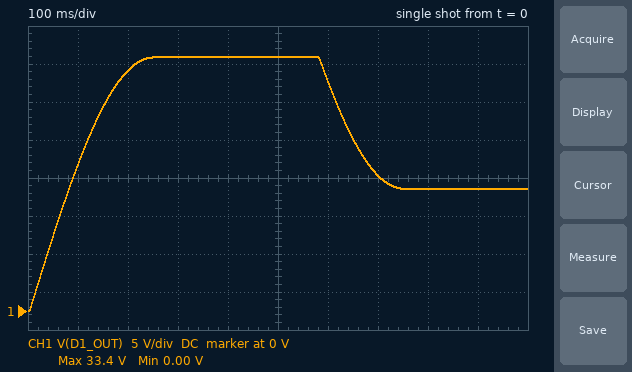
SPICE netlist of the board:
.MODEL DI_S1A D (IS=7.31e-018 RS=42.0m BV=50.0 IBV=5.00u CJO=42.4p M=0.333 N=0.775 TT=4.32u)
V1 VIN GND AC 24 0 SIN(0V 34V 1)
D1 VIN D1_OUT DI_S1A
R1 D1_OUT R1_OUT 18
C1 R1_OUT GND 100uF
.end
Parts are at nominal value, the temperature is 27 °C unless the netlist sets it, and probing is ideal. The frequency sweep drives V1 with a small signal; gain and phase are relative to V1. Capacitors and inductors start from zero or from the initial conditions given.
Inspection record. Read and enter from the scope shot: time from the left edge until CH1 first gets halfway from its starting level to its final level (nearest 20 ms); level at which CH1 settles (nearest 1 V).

40 ms
16 V
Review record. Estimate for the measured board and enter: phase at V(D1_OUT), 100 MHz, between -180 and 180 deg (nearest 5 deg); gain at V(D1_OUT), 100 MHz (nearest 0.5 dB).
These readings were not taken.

65 deg
-7.5 dB
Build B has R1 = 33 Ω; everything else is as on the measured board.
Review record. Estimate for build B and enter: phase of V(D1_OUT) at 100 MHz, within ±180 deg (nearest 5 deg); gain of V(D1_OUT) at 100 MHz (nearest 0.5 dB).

50 deg
-3.5 dB
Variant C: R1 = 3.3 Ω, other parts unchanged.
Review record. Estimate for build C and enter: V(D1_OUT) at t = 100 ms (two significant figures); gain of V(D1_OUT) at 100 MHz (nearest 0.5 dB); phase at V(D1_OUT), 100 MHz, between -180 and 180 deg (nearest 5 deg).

19 V
-21.0 dB
85 deg
